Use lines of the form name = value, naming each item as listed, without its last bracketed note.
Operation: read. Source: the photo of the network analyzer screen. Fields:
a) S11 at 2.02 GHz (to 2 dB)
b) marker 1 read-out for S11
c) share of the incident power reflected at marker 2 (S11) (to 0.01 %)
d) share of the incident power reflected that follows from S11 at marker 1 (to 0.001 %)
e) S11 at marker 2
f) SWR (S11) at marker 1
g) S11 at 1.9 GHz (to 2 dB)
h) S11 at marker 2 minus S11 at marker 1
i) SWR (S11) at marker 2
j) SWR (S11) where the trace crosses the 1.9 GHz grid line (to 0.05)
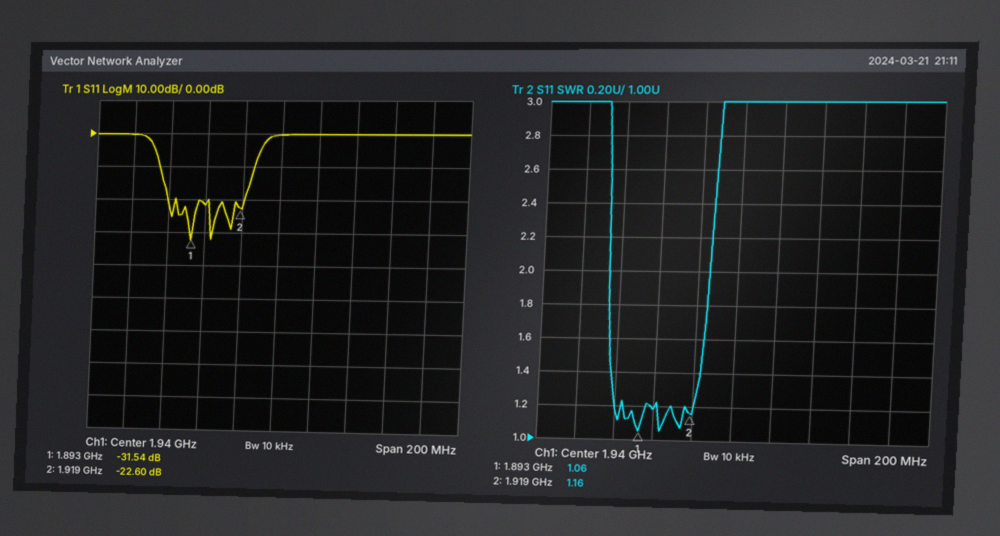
S11 at 2.02 GHz = 0 dB
marker 1 read-out for S11 = -31.54 dB
share of the incident power reflected at marker 2 (S11) = 0.55 %
share of the incident power reflected that follows from S11 at marker 1 = 0.070 %
S11 at marker 2 = -22.60 dB
SWR (S11) at marker 1 = 1.06
S11 at 1.9 GHz = -22 dB
S11 at marker 2 minus S11 at marker 1 = 8.94 dB
SWR (S11) at marker 2 = 1.16
SWR (S11) where the trace crosses the 1.9 GHz grid line = 1.20
